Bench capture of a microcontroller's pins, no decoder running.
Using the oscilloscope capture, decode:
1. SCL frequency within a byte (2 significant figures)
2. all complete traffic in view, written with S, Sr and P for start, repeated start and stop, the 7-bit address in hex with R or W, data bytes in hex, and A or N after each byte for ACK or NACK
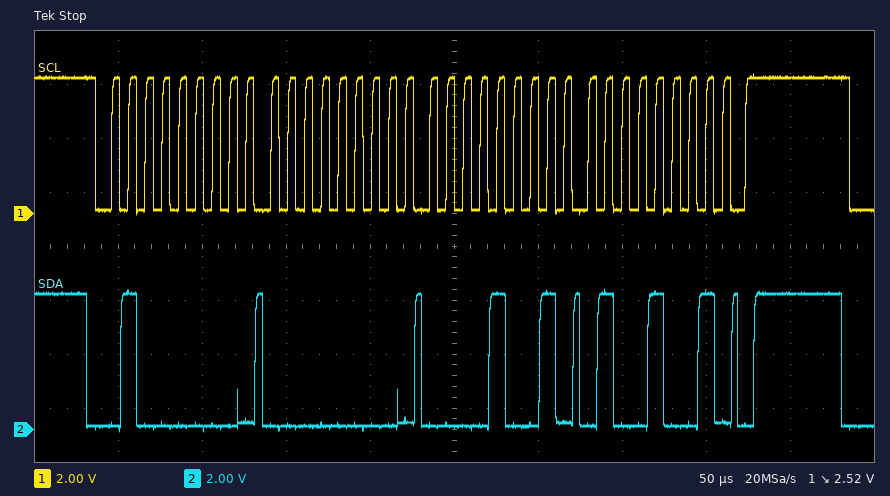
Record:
100 kHz
S 20W A 00 A 09 A 49 A P
